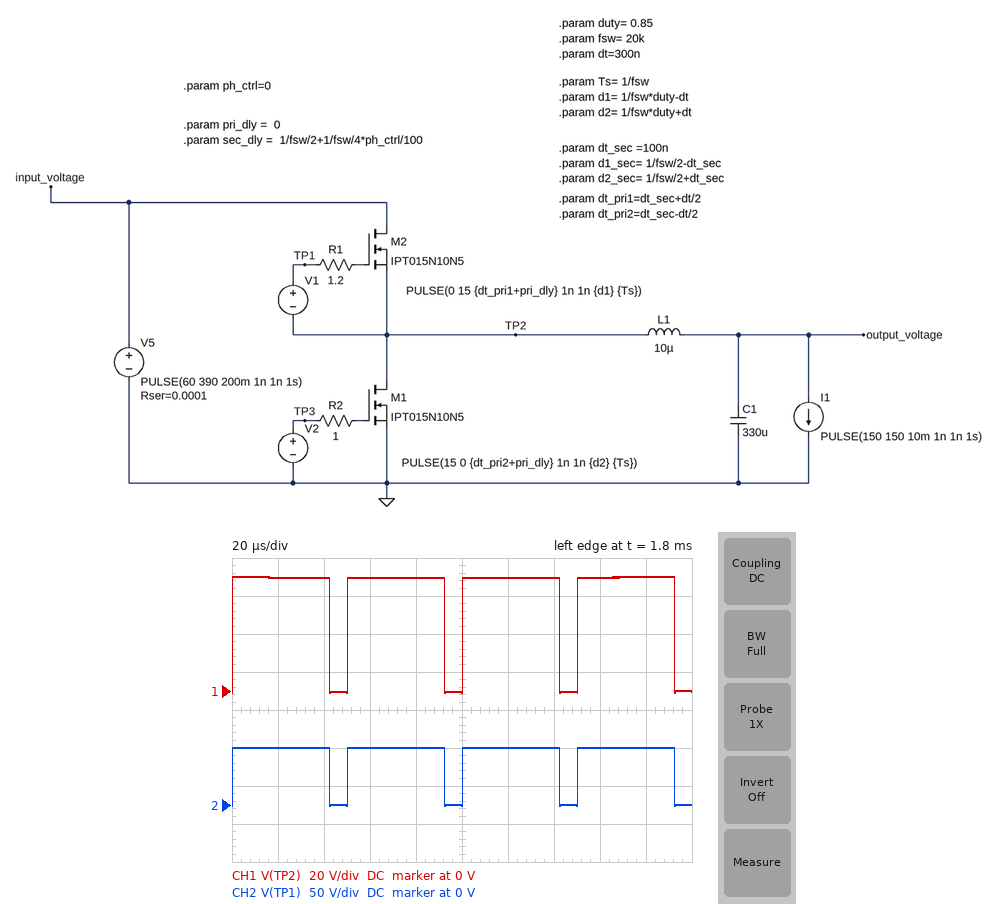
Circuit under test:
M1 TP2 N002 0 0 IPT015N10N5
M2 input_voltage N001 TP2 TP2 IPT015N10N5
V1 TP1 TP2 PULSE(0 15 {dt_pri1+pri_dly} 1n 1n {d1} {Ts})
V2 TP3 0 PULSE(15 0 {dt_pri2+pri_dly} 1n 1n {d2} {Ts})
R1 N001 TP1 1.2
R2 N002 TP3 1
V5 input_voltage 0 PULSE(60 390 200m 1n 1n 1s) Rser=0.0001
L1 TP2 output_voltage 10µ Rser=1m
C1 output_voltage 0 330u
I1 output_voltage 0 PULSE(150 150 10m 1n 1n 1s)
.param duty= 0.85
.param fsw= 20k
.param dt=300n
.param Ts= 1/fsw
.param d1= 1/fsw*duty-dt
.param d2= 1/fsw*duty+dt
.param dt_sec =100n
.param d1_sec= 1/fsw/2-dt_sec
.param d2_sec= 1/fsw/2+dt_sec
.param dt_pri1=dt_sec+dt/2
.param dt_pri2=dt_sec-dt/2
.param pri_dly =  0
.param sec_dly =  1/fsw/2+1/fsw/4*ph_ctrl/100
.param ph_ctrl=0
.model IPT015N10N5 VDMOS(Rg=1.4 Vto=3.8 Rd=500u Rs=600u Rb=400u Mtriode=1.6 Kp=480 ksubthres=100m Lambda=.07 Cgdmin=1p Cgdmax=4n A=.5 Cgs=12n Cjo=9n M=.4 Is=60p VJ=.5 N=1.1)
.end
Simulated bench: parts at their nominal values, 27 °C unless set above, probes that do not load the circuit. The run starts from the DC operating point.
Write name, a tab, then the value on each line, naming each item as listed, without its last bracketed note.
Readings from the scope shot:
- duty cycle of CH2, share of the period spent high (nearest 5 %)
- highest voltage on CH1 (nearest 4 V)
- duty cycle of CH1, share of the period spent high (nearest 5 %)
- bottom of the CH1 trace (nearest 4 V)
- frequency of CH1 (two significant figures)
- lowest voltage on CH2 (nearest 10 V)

duty cycle of CH2, share of the period spent high	85 %
highest voltage on CH1	60 V
duty cycle of CH1, share of the period spent high	85 %
bottom of the CH1 trace	0 V
frequency of CH1	20 kHz
lowest voltage on CH2	0 V
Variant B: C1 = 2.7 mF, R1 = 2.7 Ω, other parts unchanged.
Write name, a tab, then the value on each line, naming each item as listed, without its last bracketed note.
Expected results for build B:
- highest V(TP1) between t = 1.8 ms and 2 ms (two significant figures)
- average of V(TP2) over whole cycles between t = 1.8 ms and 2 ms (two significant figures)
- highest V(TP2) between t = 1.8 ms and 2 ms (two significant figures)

highest V(TP1) between t = 1.8 ms and 2 ms	76 V
average of V(TP2) over whole cycles between t = 1.8 ms and 2 ms	52 V
highest V(TP2) between t = 1.8 ms and 2 ms	61 V
